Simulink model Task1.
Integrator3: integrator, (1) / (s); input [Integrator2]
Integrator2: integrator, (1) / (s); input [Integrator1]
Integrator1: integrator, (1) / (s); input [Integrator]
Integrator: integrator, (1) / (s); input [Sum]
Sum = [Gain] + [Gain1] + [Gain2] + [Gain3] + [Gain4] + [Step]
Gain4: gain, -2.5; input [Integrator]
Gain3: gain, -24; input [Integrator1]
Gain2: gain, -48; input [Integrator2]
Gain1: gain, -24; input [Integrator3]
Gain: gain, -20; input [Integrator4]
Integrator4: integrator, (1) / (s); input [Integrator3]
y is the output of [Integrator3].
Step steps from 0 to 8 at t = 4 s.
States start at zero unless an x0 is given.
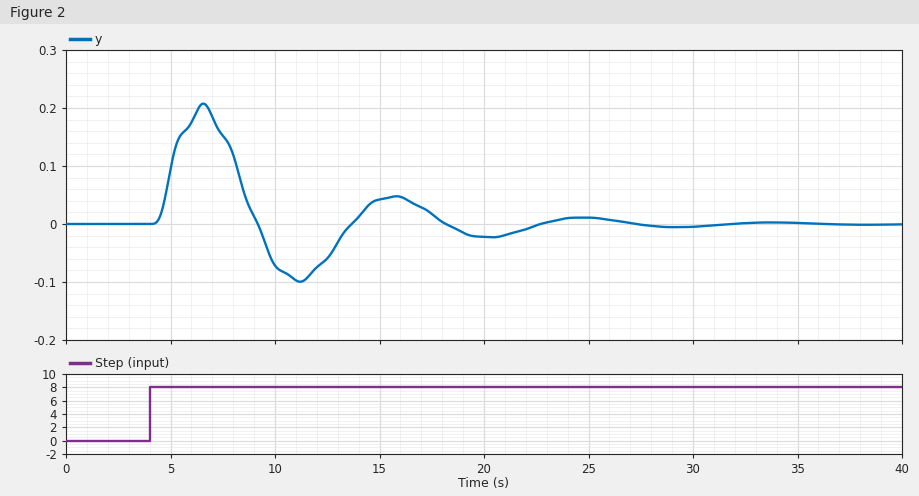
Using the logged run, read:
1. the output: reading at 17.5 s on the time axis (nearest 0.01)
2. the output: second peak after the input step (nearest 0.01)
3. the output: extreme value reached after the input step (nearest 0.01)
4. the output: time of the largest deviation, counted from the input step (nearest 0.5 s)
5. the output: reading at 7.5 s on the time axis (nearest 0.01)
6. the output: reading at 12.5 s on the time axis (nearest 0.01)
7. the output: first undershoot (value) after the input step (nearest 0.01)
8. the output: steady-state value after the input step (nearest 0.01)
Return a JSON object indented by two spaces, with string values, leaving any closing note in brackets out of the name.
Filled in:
{
  "the output: reading at 17.5 s on the time axis": "0.02",
  "the output: second peak after the input step": "0.05",
  "the output: extreme value reached after the input step": "0.21",
  "the output: time of the largest deviation, counted from the input step": "2.5 s",
  "the output: reading at 7.5 s on the time axis": "0.15",
  "the output: reading at 12.5 s on the time axis": "-0.06",
  "the output: first undershoot (value) after the input step": "-0.10",
  "the output: steady-state value after the input step": "0.00"
}
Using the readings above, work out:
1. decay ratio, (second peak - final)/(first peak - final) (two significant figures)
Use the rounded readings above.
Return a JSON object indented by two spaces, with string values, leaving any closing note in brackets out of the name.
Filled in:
{
  "decay ratio, (second peak - final)/(first peak - final)": "0.24"
}
